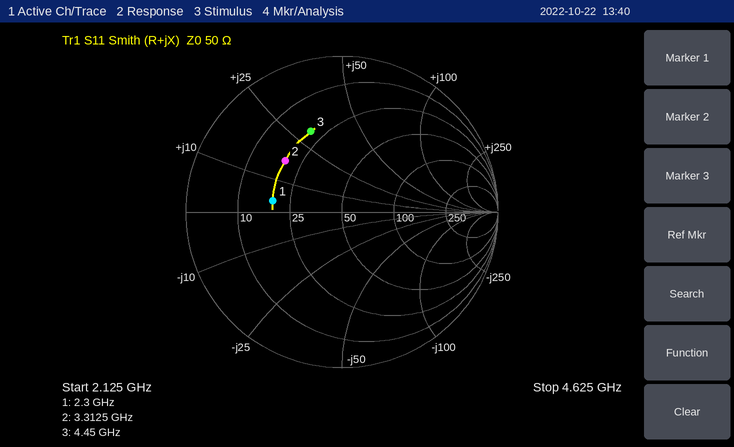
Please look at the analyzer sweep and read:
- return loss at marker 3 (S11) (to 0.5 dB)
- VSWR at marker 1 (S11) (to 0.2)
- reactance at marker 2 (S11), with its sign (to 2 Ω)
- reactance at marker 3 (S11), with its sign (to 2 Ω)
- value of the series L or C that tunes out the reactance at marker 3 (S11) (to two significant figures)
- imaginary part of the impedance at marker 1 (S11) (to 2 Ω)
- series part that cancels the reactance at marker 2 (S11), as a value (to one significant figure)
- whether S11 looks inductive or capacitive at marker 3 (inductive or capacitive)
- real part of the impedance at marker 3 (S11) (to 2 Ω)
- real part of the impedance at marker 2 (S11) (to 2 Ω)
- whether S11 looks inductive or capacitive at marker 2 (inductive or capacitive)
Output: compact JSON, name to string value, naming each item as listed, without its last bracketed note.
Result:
{"return loss at marker 3 (S11)": "5.0 dB", "VSWR at marker 1 (S11)": "2.6", "reactance at marker 2 (S11), with its sign": "+16 Ω", "reactance at marker 3 (S11), with its sign": "+30 Ω", "value of the series L or C that tunes out the reactance at marker 3 (S11)": "1.2 pF", "imaginary part of the impedance at marker 1 (S11)": "+4 Ω", "series part that cancels the reactance at marker 2 (S11), as a value": "3 pF", "whether S11 looks inductive or capacitive at marker 3": "inductive", "real part of the impedance at marker 3 (S11)": "20 Ω", "real part of the impedance at marker 2 (S11)": "20 Ω", "whether S11 looks inductive or capacitive at marker 2": "inductive"}
